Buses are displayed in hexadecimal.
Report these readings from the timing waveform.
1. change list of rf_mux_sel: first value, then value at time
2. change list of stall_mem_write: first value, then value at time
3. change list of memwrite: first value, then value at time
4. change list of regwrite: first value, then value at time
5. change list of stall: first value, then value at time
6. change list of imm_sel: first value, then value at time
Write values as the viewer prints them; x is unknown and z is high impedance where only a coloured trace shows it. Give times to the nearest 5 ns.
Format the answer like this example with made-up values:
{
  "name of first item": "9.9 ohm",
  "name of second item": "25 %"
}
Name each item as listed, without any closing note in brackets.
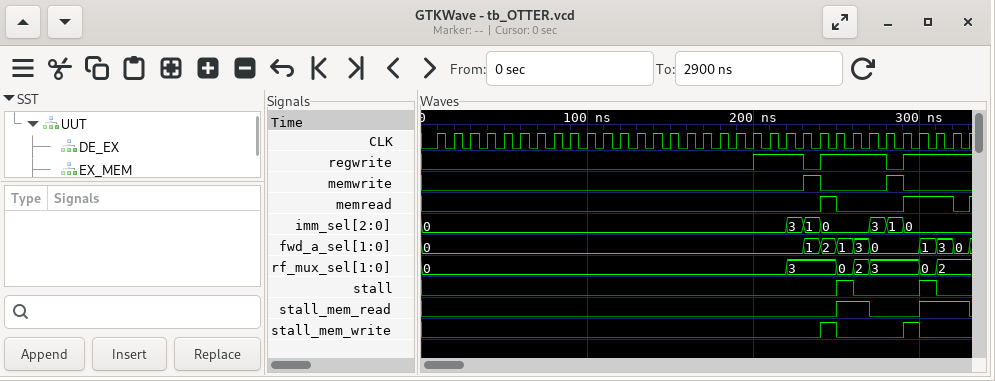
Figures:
{
  "change list of rf_mux_sel: first value, then value at time": "0, 3 at 220 ns, 0 at 250 ns, 2 at 260 ns, 3 at 270 ns, 0 at 300 ns, 2 at 310 ns",
  "change list of stall_mem_write: first value, then value at time": "0, 1 at 240 ns, 0 at 250 ns, 1 at 290 ns, 0 at 300 ns",
  "change list of memwrite: first value, then value at time": "0, 1 at 230 ns, 0 at 240 ns, 1 at 280 ns, 0 at 290 ns",
  "change list of regwrite: first value, then value at time": "0, 1 at 200 ns, 0 at 230 ns, 1 at 240 ns, 0 at 280 ns, 1 at 290 ns",
  "change list of stall: first value, then value at time": "0, 1 at 250 ns, 0 at 260 ns, 1 at 300 ns, 0 at 310 ns",
  "change list of imm_sel: first value, then value at time": "0, 3 at 220 ns, 1 at 230 ns, 0 at 240 ns, 3 at 270 ns, 1 at 280 ns, 0 at 290 ns"
}
